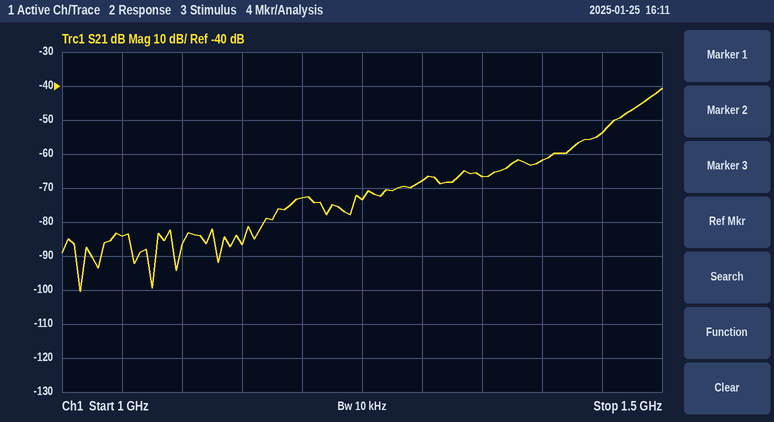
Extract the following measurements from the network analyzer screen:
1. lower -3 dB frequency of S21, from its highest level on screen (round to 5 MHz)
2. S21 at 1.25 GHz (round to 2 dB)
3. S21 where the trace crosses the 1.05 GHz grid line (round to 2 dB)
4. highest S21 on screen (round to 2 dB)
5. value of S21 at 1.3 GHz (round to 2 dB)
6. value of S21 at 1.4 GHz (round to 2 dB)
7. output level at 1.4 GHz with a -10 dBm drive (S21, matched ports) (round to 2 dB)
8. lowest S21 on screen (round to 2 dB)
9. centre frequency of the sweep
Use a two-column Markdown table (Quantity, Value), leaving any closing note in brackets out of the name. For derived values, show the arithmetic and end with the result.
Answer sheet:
| Quantity | Value |
|---|---|
| lower -3 dB frequency of S21, from its highest level on screen | 1.490 GHz |
| S21 at 1.25 GHz | -74 dB |
| S21 where the trace crosses the 1.05 GHz grid line | -84 dB |
| highest S21 on screen | -40 dB |
| value of S21 at 1.3 GHz | -68 dB |
| value of S21 at 1.4 GHz | -62 dB |
| output level at 1.4 GHz with a -10 dBm drive (S21, matched ports) | -10 dBm + (-62 dB) = -72 dBm |
| lowest S21 on screen | -100 dB |
| centre frequency of the sweep | 1.25 GHz |
